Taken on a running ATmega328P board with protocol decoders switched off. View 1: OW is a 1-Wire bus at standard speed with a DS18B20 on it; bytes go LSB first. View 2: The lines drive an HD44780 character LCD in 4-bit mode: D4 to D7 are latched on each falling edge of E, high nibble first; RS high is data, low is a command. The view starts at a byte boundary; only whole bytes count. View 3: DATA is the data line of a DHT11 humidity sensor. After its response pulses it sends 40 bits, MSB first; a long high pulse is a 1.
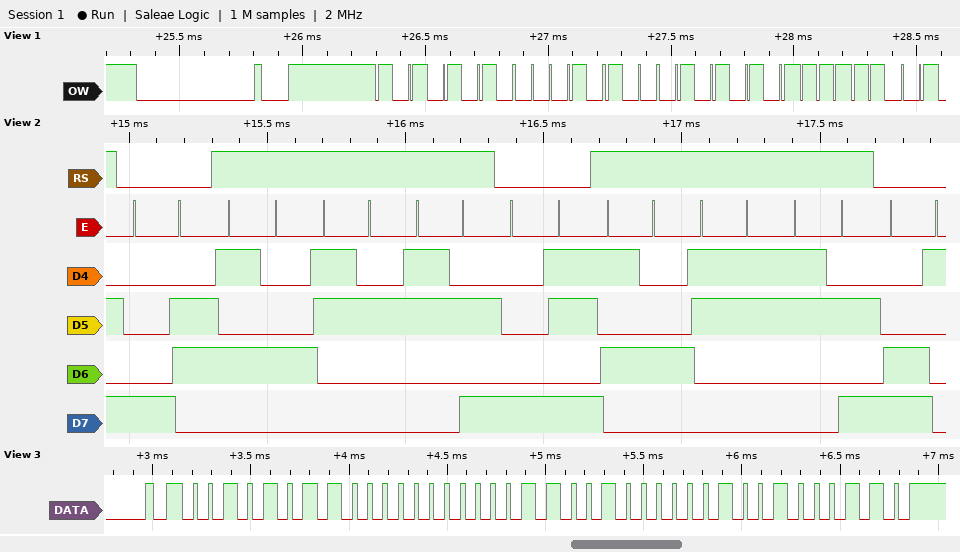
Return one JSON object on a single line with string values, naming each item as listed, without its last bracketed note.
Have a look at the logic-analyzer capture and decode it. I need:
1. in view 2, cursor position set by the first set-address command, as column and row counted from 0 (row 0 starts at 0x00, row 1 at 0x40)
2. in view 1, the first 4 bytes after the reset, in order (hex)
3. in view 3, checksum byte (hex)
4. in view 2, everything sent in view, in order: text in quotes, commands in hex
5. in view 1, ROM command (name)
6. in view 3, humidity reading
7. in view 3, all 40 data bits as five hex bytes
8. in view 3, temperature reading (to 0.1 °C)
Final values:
{"in view 2, cursor position set by the first set-address command, as column and row counted from 0": "column 6, row 0", "in view 1, the first 4 bytes after the reset, in order": "55 28 AA 9F", "in view 3, checksum byte": "0x46", "in view 2, everything sent in view, in order: text in quotes, commands in hex": "0x86 \"T2:\" 0x8B \"T3:\" 0xC1", "in view 1, ROM command": "Match ROM", "in view 3, humidity reading": "43 %", "in view 3, all 40 data bits as five hex bytes": "2B 00 19 02 46", "in view 3, temperature reading": "25.2 °C"}
